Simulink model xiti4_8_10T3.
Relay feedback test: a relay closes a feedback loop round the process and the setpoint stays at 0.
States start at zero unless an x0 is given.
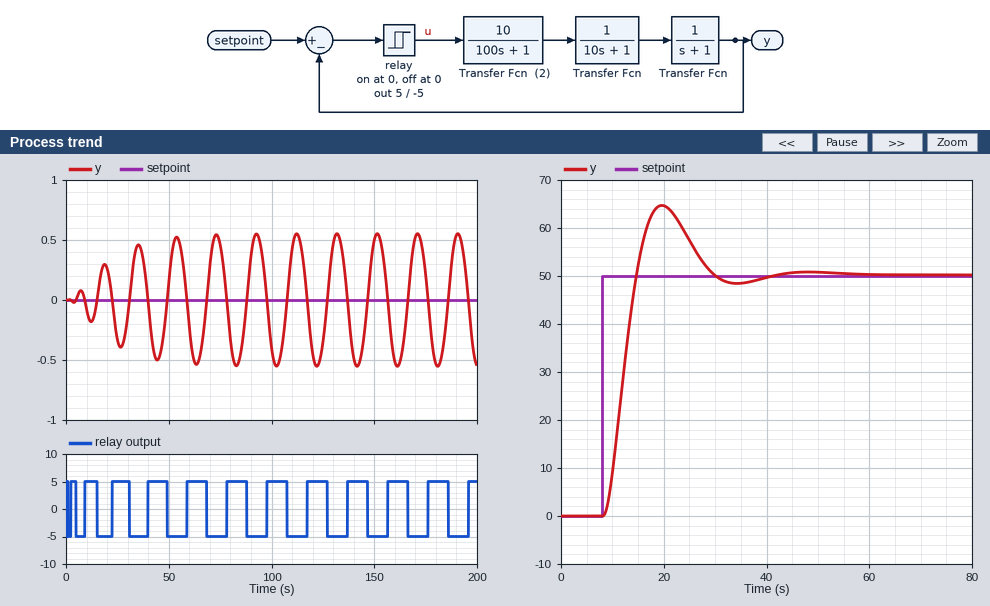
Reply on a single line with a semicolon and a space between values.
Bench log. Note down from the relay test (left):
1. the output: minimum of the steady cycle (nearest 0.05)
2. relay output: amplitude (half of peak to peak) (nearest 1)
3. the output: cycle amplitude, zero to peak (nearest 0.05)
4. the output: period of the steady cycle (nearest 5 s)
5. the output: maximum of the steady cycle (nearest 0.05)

-0.55; 5; 0.55; 20 s; 0.55
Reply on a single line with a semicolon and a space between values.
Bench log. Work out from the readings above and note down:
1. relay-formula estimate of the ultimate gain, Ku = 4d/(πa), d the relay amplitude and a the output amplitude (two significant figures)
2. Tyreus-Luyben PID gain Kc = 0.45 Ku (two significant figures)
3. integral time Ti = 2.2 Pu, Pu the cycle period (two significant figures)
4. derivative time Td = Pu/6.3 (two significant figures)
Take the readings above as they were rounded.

12; 5.4; 44 s; 3.2 s
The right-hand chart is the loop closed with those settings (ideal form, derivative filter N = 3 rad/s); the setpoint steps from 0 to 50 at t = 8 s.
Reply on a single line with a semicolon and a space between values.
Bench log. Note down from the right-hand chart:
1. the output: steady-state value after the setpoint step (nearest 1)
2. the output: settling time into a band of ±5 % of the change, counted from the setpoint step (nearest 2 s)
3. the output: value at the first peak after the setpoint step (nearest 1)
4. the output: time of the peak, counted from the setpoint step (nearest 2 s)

50; 20 s; 65; 12 s
